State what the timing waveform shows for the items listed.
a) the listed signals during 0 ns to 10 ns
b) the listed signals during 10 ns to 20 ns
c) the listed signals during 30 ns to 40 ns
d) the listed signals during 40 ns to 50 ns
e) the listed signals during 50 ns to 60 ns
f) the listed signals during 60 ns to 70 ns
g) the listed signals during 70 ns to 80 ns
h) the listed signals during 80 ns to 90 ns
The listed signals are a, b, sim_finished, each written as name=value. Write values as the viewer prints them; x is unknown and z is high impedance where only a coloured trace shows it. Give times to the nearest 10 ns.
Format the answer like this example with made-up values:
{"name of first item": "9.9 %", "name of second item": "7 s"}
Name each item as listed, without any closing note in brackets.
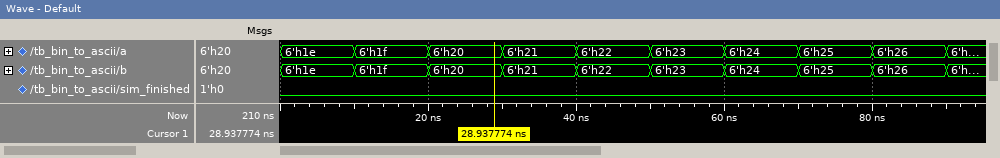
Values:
{"the listed signals during 0 ns to 10 ns": "a=6'h1e, b=6'h1e, sim_finished=0", "the listed signals during 10 ns to 20 ns": "a=6'h1f, b=6'h1f, sim_finished=0", "the listed signals during 30 ns to 40 ns": "a=6'h21, b=6'h21, sim_finished=0", "the listed signals during 40 ns to 50 ns": "a=6'h22, b=6'h22, sim_finished=0", "the listed signals during 50 ns to 60 ns": "a=6'h23, b=6'h23, sim_finished=0", "the listed signals during 60 ns to 70 ns": "a=6'h24, b=6'h24, sim_finished=0", "the listed signals during 70 ns to 80 ns": "a=6'h25, b=6'h25, sim_finished=0", "the listed signals during 80 ns to 90 ns": "a=6'h26, b=6'h26, sim_finished=0"}
